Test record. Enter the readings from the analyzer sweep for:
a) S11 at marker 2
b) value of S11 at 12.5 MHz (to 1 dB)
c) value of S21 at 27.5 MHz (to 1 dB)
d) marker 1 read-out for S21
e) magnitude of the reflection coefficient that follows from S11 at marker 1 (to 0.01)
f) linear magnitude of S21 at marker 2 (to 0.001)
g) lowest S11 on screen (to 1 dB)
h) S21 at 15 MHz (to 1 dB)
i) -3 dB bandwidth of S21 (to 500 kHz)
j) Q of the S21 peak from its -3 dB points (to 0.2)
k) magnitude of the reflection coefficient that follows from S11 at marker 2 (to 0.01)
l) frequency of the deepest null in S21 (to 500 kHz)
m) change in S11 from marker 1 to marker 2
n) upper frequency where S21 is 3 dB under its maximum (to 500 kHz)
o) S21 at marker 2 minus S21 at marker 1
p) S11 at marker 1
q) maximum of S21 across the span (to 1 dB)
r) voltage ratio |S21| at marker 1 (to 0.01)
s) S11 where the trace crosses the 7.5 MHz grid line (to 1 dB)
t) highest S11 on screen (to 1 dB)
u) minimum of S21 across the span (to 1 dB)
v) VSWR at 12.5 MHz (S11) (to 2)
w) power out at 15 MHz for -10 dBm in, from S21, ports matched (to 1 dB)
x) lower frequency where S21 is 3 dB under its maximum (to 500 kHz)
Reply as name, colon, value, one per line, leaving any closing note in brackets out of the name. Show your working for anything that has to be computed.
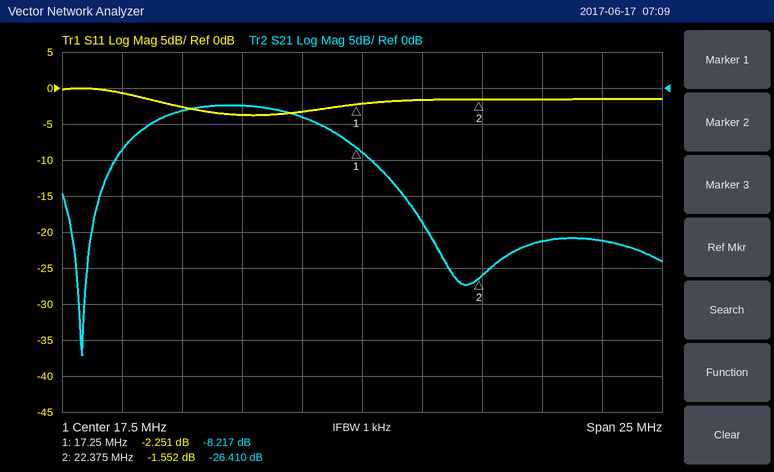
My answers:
S11 at marker 2: -1.552 dB
value of S11 at 12.5 MHz: -4 dB
value of S21 at 27.5 MHz: -21 dB
marker 1 read-out for S21: -8.217 dB
magnitude of the reflection coefficient that follows from S11 at marker 1: 10^(-2.251/20) ≈ 0.77
linear magnitude of S21 at marker 2: 10^(-26.41/20) ≈ 0.048
lowest S11 on screen: -4 dB
S21 at 15 MHz: -4 dB
-3 dB bandwidth of S21: 16.0 MHz − 8.5 MHz = 7.5 MHz
Q of the S21 peak from its -3 dB points: 12.25 MHz / 7.5 MHz ≈ 1.6
magnitude of the reflection coefficient that follows from S11 at marker 2: 10^(-1.552/20) ≈ 0.84
frequency of the deepest null in S21: 6.0 MHz
change in S11 from marker 1 to marker 2: -1.552 − (-2.251) = 0.699 dB
upper frequency where S21 is 3 dB under its maximum: 16.0 MHz
S21 at marker 2 minus S21 at marker 1: -26.41 − (-8.217) = -18.193 dB
S11 at marker 1: -2.251 dB
maximum of S21 across the span: -2 dB
voltage ratio |S21| at marker 1: 10^(-8.217/20) ≈ 0.39
S11 where the trace crosses the 7.5 MHz grid line: -1 dB
highest S11 on screen: 0 dB
minimum of S21 across the span: -37 dB
VSWR at 12.5 MHz (S11): |Γ| = 10^(-4/20) = 0.6310; VSWR = (1 + 0.6310)/(1 − 0.6310) ≈ 4
power out at 15 MHz for -10 dBm in, from S21, ports matched: -10 dBm + (-4 dB) = -14 dBm
lower frequency where S21 is 3 dB under its maximum: 8.5 MHz
